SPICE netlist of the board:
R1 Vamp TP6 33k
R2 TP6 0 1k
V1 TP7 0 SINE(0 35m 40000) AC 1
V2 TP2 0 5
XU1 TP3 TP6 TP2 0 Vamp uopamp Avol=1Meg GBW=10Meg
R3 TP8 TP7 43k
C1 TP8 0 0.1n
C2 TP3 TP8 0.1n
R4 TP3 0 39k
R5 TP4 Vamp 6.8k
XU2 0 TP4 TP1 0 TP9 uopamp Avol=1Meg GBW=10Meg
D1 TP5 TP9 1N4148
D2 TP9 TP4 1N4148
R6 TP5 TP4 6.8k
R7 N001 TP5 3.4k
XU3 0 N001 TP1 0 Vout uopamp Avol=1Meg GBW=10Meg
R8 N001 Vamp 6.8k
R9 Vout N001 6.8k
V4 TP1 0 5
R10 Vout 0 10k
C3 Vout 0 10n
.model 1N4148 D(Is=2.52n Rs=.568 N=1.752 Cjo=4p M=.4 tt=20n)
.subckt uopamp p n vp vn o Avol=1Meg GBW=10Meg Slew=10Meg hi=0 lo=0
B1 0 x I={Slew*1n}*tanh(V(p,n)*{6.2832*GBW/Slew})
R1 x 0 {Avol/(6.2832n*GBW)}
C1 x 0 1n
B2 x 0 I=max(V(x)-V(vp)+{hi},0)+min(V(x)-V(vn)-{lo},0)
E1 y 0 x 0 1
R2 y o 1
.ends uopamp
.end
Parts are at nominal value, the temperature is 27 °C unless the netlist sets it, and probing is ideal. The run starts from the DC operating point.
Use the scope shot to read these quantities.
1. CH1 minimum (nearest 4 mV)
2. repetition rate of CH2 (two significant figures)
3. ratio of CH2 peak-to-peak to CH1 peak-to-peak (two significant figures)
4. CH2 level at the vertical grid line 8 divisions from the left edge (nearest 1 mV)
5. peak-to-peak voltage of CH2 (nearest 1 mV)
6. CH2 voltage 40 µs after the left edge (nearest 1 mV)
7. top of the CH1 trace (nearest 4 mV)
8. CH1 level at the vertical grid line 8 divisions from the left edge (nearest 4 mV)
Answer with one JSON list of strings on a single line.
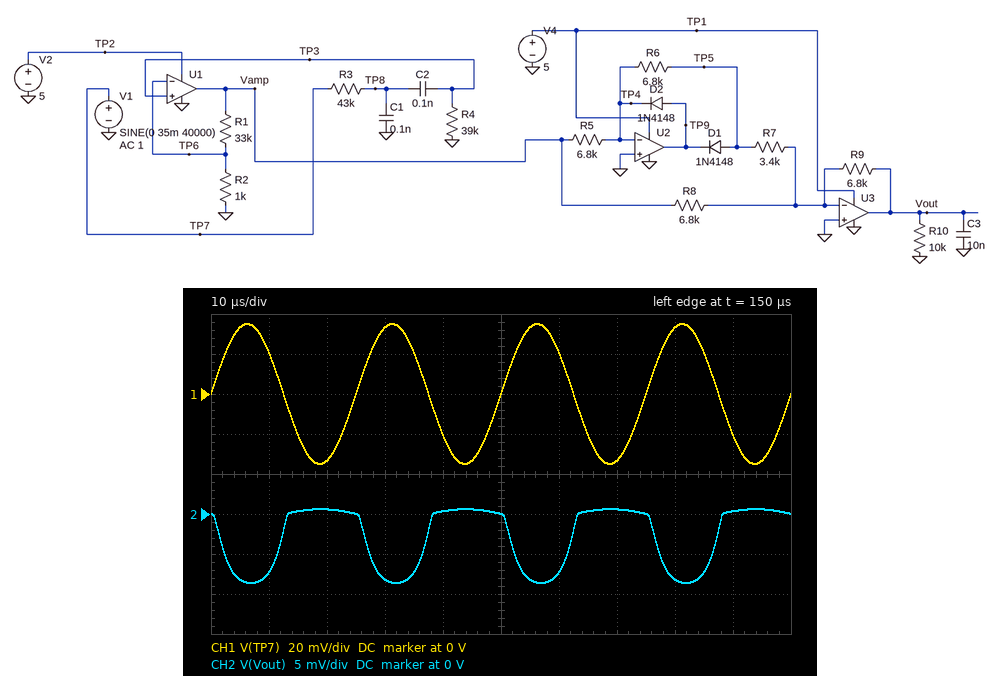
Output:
["-36 mV", "40 kHz", "0.13", "-8 mV", "9 mV", "0 V", "36 mV", "32 mV"]
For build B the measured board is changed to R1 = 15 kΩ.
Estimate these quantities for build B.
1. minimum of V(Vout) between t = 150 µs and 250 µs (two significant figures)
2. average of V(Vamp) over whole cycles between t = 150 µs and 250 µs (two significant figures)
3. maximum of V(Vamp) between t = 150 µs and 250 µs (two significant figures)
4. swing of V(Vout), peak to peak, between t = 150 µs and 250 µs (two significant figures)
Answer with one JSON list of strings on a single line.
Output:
["-5.5 mV", "55 mV", "170 mV", "6.1 mV"]
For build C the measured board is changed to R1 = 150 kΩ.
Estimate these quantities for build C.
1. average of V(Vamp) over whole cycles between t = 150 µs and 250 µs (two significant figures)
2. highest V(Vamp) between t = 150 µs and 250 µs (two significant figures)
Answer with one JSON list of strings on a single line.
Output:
["490 mV", "1.4 V"]
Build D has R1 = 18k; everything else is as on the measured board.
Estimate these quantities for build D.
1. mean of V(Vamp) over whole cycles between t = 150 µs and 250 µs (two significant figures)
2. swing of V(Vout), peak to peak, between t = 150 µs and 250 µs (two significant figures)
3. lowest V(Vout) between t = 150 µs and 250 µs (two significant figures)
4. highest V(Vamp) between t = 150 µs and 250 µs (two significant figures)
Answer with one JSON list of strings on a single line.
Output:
["66 mV", "6.9 mV", "-6.3 mV", "210 mV"]
